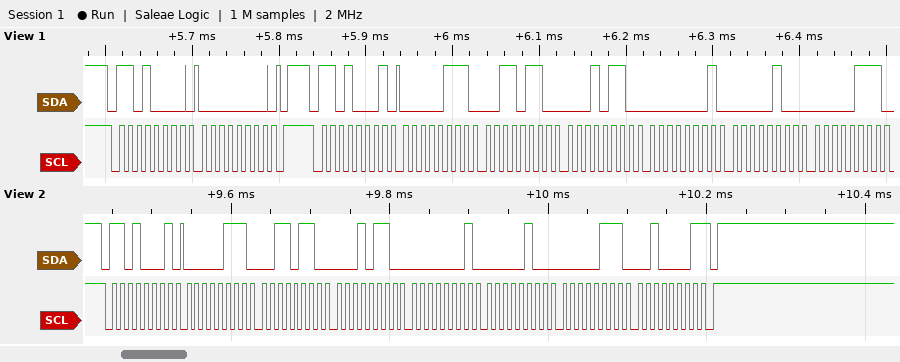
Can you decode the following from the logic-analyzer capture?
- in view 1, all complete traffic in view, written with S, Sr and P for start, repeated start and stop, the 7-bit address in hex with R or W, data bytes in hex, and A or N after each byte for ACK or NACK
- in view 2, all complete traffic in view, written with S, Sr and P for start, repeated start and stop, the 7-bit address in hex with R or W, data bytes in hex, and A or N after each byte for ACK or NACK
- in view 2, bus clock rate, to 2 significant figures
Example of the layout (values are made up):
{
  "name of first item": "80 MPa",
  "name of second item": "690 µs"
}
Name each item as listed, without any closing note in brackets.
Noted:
{
  "in view 1, all complete traffic in view, written with S, Sr and P for start, repeated start and stop, the 7-bit address in hex with R or W, data bytes in hex, and A or N after each byte for ACK or NACK": "S 68W A 00 A P S 68R A 07 A 36 A 16 A 01 A 04 A 07 A",
  "in view 2, all complete traffic in view, written with S, Sr and P for start, repeated start and stop, the 7-bit address in hex with R or W, data bytes in hex, and A or N after each byte for ACK or NACK": "S 68R A 07 A 36 A 16 A 01 A 04 A 07 A 21 N P",
  "in view 2, bus clock rate, to 2 significant figures": "100 kHz"
}
